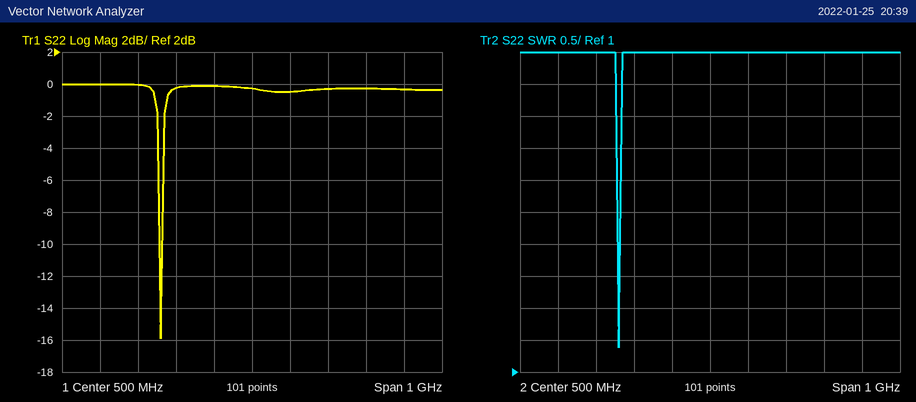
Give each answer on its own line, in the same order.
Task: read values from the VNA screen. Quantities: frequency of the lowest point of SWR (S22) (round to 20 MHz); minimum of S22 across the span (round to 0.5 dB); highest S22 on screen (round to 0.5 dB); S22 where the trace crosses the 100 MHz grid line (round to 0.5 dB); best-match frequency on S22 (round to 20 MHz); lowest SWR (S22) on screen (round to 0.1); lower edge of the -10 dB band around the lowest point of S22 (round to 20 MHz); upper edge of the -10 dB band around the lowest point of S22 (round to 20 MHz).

260 MHz
-16.0 dB
0.0 dB
0.0 dB
260 MHz
1.4
260 MHz
260 MHz
